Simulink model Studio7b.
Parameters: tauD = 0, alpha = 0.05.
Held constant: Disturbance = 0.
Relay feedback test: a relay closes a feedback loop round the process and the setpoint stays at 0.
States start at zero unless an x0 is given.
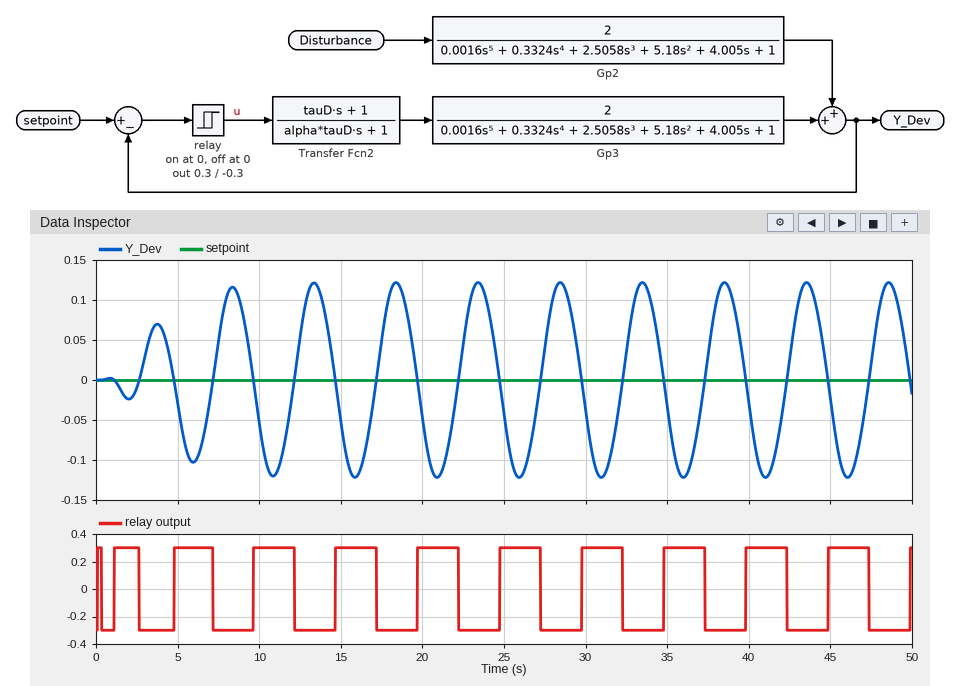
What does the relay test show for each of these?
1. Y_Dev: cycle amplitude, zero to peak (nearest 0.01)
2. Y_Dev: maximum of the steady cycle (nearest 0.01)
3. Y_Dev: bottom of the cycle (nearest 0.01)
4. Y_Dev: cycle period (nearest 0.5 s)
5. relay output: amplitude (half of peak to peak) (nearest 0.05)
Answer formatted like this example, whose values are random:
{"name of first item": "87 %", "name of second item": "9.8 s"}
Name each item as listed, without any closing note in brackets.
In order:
{"Y_Dev: cycle amplitude, zero to peak": "0.12", "Y_Dev: maximum of the steady cycle": "0.12", "Y_Dev: bottom of the cycle": "-0.12", "Y_Dev: cycle period": "5.0 s", "relay output: amplitude (half of peak to peak)": "0.30"}
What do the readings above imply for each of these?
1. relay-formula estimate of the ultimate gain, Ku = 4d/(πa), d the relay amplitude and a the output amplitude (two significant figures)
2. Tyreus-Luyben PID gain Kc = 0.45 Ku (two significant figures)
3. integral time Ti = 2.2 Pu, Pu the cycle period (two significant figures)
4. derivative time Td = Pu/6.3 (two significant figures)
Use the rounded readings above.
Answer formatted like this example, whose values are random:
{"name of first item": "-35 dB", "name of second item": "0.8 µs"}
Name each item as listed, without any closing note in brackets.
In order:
{"relay-formula estimate of the ultimate gain, Ku = 4d/(πa), d the relay amplitude and a the output amplitude": "3.2", "Tyreus-Luyben PID gain Kc = 0.45 Ku": "1.4", "integral time Ti = 2.2 Pu, Pu the cycle period": "11 s", "derivative time Td = Pu/6.3": "0.79 s"}
